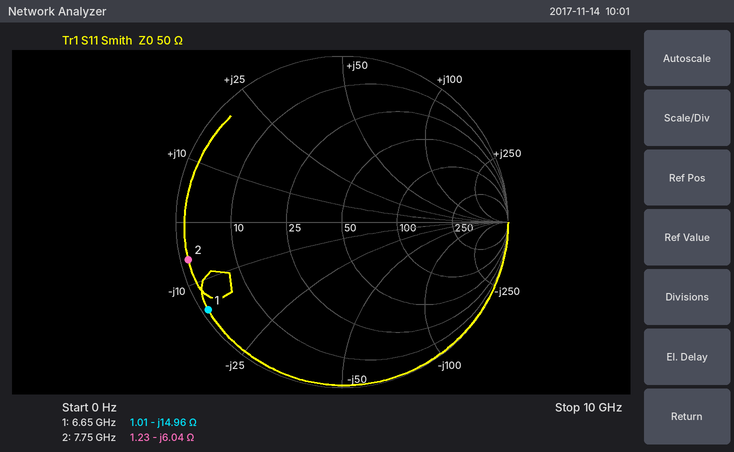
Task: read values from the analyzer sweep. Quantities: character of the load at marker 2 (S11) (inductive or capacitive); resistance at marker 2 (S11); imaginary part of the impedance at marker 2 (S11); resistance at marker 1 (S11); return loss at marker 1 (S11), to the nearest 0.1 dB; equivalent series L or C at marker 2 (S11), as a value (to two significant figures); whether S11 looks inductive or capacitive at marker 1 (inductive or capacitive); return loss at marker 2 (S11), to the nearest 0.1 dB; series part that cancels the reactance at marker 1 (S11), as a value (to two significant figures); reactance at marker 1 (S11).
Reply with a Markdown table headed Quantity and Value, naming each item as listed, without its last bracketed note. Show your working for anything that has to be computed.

| Quantity | Value |
|---|---|
| character of the load at marker 2 (S11) | capacitive |
| resistance at marker 2 | 1.23 Ω |
| imaginary part of the impedance at marker 2 | -6.04 Ω |
| resistance at marker 1 | 1.01 Ω |
| return loss at marker 1 (S11), to the nearest 0.1 dB | 0.3 dB |
| equivalent series L or C at marker 2 (S11), as a value | C = 1/(2π × 7.75 GHz × 6.04 Ω) ≈ 3.4 pF |
| whether S11 looks inductive or capacitive at marker 1 | capacitive |
| return loss at marker 2 (S11), to the nearest 0.1 dB | 0.4 dB |
| series part that cancels the reactance at marker 1 (S11), as a value | L = 14.96 Ω/(2π × 6.65 GHz) ≈ 358 pH, so 360 pH to two significant figures |
| reactance at marker 1 | -14.96 Ω |
